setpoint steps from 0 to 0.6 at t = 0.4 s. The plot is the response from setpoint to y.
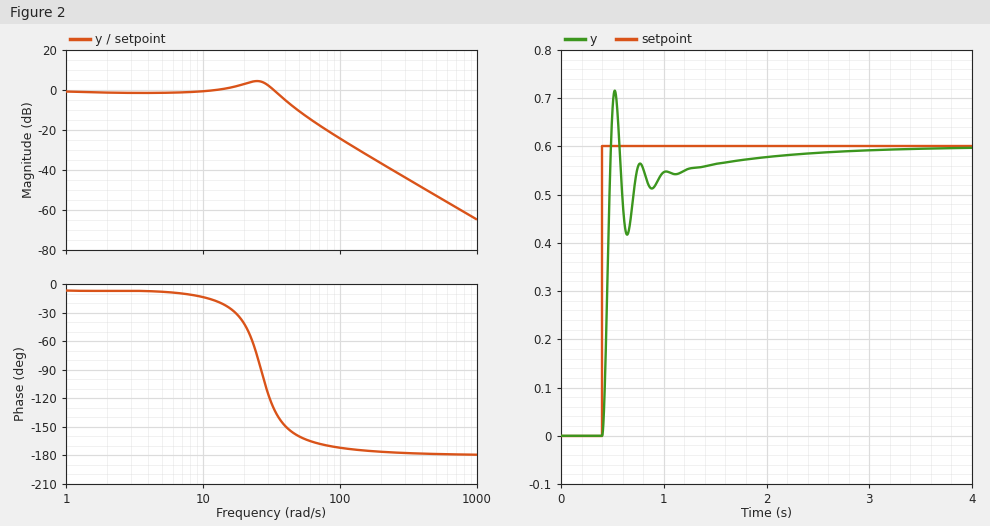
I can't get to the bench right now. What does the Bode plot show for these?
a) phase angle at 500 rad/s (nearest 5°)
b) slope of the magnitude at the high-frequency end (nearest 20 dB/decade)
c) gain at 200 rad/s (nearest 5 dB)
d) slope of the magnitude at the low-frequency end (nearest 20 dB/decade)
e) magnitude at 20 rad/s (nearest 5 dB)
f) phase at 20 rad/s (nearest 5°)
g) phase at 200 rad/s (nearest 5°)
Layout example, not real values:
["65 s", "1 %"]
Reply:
["-180°", "-40 dB/decade", "-35 dB", "0 dB/decade", "5 dB", "-40°", "-175°"]
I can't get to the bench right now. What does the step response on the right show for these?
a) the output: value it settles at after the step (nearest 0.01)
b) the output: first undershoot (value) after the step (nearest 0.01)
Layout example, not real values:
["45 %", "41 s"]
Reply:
["0.60", "0.42"]
